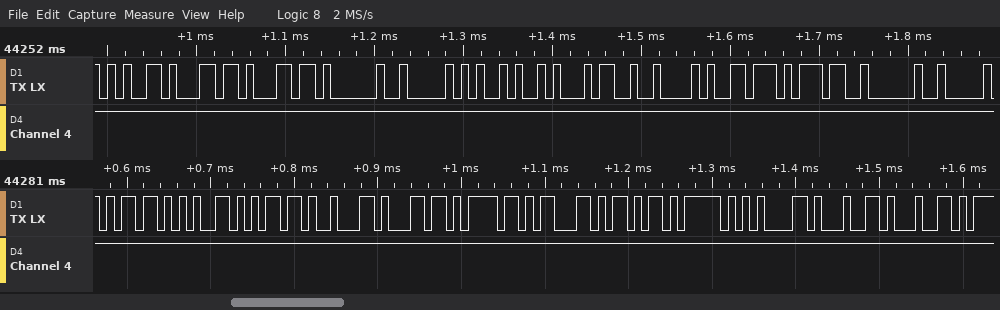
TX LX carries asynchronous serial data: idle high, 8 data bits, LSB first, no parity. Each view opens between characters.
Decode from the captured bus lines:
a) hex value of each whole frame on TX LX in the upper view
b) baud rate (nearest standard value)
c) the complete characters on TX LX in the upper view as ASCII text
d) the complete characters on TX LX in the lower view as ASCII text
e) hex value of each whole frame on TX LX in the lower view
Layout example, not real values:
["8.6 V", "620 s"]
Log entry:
["65, 6C, 6C, 20, 50, 4A, 34, 42, 76, 37, 20", "115200 baud", "\"ell PJ4Bv7 \"", "\"memblock_add\"", "6D, 65, 6D, 62, 6C, 6F, 63, 6B, 5F, 61, 64, 64"]
